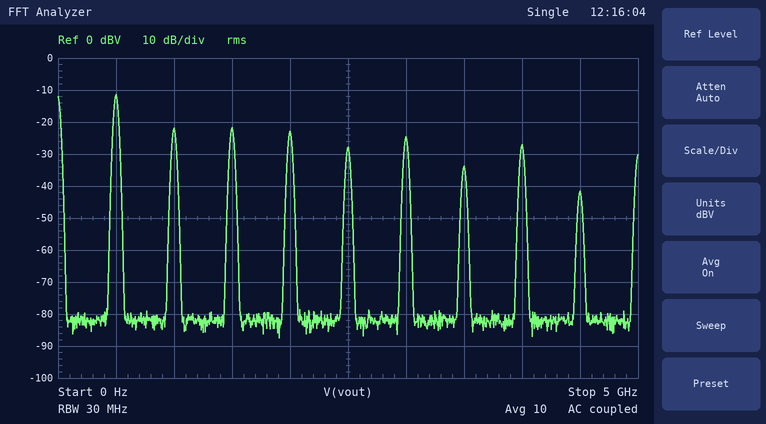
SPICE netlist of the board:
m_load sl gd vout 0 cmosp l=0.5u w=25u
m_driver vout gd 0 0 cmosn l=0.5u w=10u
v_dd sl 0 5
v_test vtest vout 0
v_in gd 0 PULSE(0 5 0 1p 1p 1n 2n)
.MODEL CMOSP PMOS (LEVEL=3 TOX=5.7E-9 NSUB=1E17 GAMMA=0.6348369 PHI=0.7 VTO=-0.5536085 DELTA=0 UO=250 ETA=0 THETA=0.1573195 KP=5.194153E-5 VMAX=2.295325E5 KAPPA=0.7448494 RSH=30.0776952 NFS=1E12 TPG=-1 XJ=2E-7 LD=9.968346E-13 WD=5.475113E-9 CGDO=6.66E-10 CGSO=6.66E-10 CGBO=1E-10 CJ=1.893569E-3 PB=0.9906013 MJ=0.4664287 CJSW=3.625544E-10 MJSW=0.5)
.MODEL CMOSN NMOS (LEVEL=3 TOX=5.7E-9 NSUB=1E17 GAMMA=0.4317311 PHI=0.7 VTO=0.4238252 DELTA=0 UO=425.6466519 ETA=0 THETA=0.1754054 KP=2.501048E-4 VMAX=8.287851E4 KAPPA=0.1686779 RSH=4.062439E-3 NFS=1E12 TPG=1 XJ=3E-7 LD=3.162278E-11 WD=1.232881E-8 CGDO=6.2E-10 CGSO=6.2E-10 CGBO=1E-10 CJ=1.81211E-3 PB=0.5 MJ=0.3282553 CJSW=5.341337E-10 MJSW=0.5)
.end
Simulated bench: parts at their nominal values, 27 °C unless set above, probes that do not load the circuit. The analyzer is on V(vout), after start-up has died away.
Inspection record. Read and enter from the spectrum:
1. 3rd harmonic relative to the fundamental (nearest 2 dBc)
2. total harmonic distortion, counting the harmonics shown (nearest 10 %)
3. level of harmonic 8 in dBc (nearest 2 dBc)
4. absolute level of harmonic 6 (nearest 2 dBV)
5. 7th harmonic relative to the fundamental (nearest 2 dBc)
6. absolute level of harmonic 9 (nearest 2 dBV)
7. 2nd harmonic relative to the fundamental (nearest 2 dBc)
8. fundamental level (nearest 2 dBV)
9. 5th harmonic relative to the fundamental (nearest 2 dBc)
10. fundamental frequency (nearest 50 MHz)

-10 dBc
60 %
-16 dBc
-24 dBV
-22 dBc
-42 dBV
-10 dBc
-12 dBV
-16 dBc
500 MHz
